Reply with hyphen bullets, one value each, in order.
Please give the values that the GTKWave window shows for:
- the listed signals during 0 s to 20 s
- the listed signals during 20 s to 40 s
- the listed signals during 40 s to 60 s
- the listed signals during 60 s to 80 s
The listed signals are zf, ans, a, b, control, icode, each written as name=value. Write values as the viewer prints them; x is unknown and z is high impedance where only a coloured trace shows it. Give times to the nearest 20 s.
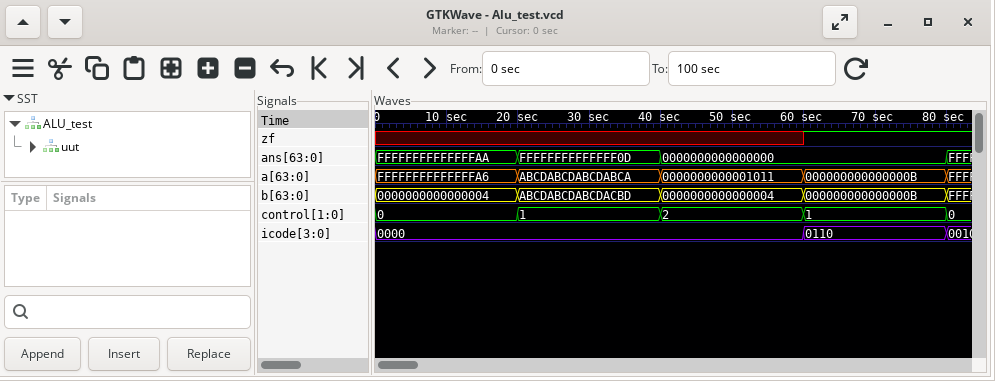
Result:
- zf=x, ans=FFFFFFFFFFFFFFAA, a=FFFFFFFFFFFFFFA6, b=0000000000000004, control=0, icode=0000
- zf=x, ans=FFFFFFFFFFFFFF0D, a=ABCDABCDABCDABCA, b=ABCDABCDABCDACBD, control=1, icode=0000
- zf=x, ans=0000000000000000, a=0000000000001011, b=0000000000000004, control=2, icode=0000
- zf=1, ans=0000000000000000, a=000000000000000B, b=000000000000000B, control=1, icode=0110
